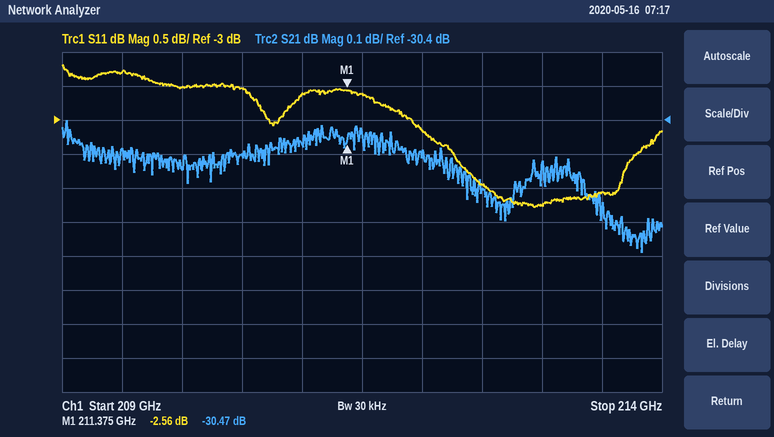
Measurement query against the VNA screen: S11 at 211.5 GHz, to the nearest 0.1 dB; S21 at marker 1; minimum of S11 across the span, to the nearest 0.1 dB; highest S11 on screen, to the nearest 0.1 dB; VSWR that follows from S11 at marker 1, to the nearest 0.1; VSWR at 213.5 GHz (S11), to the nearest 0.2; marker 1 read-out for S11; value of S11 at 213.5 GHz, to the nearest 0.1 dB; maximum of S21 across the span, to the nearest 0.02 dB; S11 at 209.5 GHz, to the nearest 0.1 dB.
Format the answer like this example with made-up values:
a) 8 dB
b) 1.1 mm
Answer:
a) -2.6 dB
b) -30.47 dB
c) -4.3 dB
d) -2.2 dB
e) 6.8
f) 4.4
g) -2.56 dB
h) -4.1 dB
i) -30.40 dB
j) -2.3 dB
